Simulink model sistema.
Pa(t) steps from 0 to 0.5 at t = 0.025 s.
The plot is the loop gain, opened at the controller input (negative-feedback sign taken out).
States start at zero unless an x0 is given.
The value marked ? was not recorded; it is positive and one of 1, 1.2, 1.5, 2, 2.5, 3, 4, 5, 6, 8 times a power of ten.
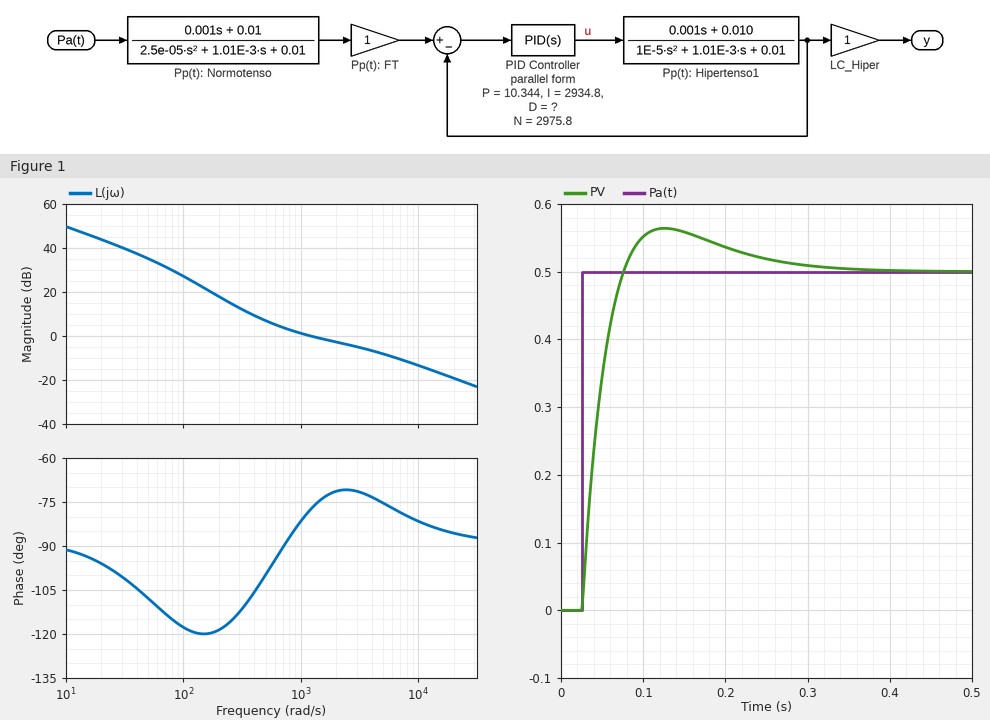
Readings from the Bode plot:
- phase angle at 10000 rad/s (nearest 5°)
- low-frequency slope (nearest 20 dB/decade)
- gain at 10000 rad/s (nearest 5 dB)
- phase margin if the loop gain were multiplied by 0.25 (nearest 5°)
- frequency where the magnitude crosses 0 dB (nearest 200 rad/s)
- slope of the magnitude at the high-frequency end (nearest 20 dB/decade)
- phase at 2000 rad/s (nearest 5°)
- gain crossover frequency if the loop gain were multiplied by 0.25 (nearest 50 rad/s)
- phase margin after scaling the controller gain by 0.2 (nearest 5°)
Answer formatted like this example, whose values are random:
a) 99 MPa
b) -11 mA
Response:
a) -80°
b) -20 dB/decade
c) -15 dB
d) 70°
e) 1200 rad/s
f) -20 dB/decade
g) -70°
h) 300 rad/s
i) 65°
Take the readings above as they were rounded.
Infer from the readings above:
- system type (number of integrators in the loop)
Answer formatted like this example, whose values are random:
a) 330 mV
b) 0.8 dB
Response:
a) 1
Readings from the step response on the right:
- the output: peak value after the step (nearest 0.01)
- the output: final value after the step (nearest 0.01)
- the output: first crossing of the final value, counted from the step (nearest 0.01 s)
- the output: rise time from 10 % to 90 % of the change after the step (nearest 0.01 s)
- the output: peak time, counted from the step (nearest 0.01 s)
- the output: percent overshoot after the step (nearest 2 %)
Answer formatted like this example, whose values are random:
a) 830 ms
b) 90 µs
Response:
a) 0.56
b) 0.50
c) 0.05 s
d) 0.04 s
e) 0.10 s
f) 12 %
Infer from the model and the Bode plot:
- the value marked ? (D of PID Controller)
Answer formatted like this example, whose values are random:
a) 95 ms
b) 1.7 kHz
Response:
a) 0.004
